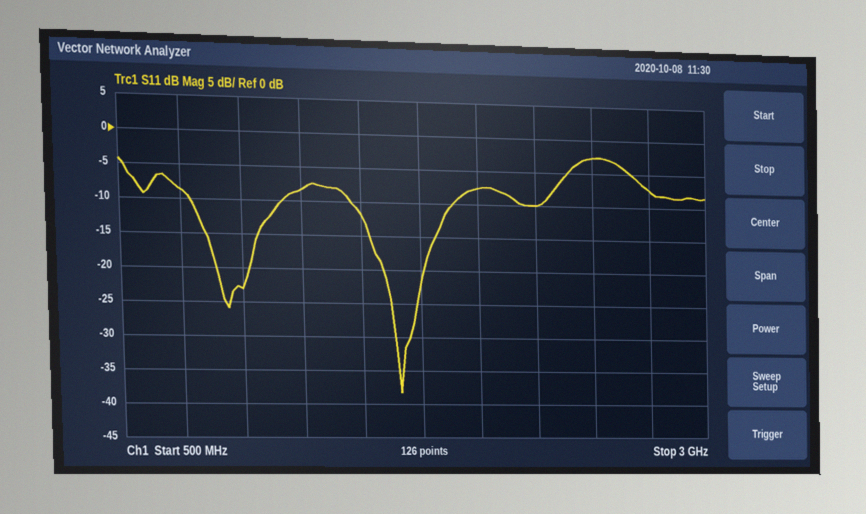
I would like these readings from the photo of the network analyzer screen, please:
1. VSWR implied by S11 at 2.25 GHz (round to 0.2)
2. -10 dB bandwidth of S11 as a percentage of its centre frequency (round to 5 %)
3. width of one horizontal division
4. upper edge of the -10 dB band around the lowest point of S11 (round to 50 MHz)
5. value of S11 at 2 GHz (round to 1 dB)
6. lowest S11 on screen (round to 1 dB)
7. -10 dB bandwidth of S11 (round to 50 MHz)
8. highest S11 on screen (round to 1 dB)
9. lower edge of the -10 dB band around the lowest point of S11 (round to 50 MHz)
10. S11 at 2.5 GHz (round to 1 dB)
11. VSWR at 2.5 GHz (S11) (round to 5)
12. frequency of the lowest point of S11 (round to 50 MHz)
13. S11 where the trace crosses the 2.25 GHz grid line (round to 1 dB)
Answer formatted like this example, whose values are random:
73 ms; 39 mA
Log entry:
2.0; 25 %; 250 MHz; 1.90 GHz; -8 dB; -38 dB; 450 MHz; -3 dB; 1.45 GHz; -3 dB; 5; 1.65 GHz; -10 dB
